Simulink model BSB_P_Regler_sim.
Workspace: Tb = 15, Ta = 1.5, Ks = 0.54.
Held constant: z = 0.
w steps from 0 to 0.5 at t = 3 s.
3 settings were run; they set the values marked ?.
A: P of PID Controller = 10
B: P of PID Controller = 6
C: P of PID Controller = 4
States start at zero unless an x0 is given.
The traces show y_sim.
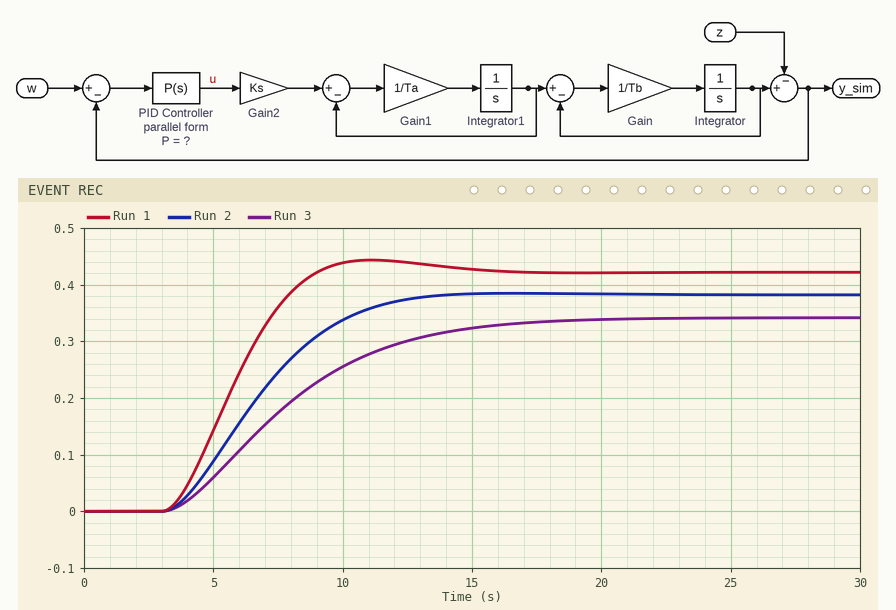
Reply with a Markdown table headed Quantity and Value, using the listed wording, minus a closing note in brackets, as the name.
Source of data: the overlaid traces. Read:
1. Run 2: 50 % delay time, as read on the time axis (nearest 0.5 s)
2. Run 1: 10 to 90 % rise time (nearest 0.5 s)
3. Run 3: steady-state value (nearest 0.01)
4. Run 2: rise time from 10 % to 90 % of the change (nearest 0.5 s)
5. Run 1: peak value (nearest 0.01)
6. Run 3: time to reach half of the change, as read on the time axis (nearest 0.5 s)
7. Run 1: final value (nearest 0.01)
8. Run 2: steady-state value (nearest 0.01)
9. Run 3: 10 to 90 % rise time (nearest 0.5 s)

| Quantity | Value |
|---|---|
| Run 2: 50 % delay time, as read on the time axis | 6.5 s |
| Run 1: 10 to 90 % rise time | 4.0 s |
| Run 3: steady-state value | 0.34 |
| Run 2: rise time from 10 % to 90 % of the change | 6.0 s |
| Run 1: peak value | 0.44 |
| Run 3: time to reach half of the change, as read on the time axis | 7.5 s |
| Run 1: final value | 0.42 |
| Run 2: steady-state value | 0.38 |
| Run 3: 10 to 90 % rise time | 8.5 s |
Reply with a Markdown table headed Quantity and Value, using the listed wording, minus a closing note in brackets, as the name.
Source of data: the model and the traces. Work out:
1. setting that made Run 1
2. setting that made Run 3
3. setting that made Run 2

| Quantity | Value |
|---|---|
| setting that made Run 1 | A |
| setting that made Run 3 | C |
| setting that made Run 2 | B |
